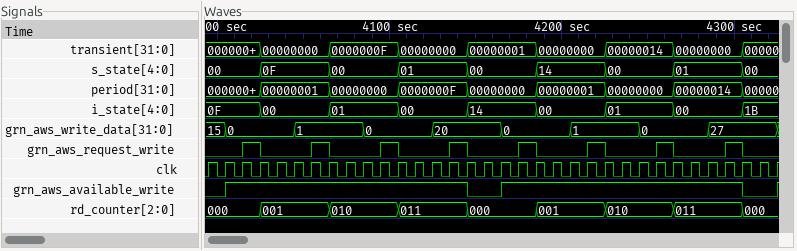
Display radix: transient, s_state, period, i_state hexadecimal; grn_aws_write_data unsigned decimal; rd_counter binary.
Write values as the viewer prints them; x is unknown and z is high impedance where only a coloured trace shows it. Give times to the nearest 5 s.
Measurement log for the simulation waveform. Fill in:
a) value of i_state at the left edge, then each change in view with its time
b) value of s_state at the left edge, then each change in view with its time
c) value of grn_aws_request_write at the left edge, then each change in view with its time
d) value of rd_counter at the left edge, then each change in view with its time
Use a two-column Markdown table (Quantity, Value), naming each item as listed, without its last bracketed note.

| Quantity | Value |
|---|---|
| value of i_state at the left edge, then each change in view with its time | 0F, 00 at 4025 s, 01 at 4065 s, 00 at 4105 s, 14 at 4145 s, 00 at 4185 s, 01 at 4225 s, 00 at 4265 s, 1B at 4305 s |
| value of s_state at the left edge, then each change in view with its time | 00, 0F at 4025 s, 00 at 4065 s, 01 at 4105 s, 00 at 4145 s, 14 at 4185 s, 00 at 4225 s, 01 at 4265 s, 00 at 4305 s |
| value of grn_aws_request_write at the left edge, then each change in view with its time | 0, 1 at 4015 s, 0 at 4025 s, 1 at 4055 s, 0 at 4065 s, 1 at 4095 s, 0 at 4105 s, 1 at 4135 s, 0 at 4145 s, 1 at 4175 s, 0 at 4185 s, 1 at 4215 s, 0 at 4225 s, 1 at 4255 s, 0 at 4265 s, 1 at 4295 s, 0 at 4305 s |
| value of rd_counter at the left edge, then each change in view with its time | 000, 001 at 4025 s, 010 at 4065 s, 011 at 4105 s, 000 at 4145 s, 001 at 4185 s, 010 at 4225 s, 011 at 4265 s, 000 at 4305 s |
